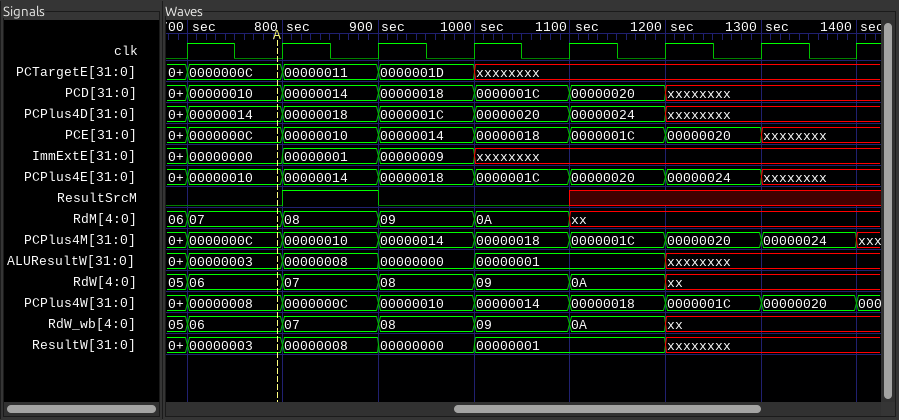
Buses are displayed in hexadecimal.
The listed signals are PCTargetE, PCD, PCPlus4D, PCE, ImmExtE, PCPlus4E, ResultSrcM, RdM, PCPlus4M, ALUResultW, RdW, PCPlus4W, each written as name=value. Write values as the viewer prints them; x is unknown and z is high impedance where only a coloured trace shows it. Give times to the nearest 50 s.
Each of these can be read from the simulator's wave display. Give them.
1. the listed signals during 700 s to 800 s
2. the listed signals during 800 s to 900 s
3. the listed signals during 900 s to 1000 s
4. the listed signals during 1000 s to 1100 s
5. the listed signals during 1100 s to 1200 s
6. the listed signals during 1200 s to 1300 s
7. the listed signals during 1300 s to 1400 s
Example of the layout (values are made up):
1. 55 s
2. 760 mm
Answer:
1. PCTargetE=0000000C, PCD=00000010, PCPlus4D=00000014, PCE=0000000C, ImmExtE=00000000, PCPlus4E=00000010, ResultSrcM=0, RdM=07, PCPlus4M=0000000C, ALUResultW=00000003, RdW=06, PCPlus4W=00000008
2. PCTargetE=00000011, PCD=00000014, PCPlus4D=00000018, PCE=00000010, ImmExtE=00000001, PCPlus4E=00000014, ResultSrcM=1, RdM=08, PCPlus4M=00000010, ALUResultW=00000008, RdW=07, PCPlus4W=0000000C
3. PCTargetE=0000001D, PCD=00000018, PCPlus4D=0000001C, PCE=00000014, ImmExtE=00000009, PCPlus4E=00000018, ResultSrcM=0, RdM=09, PCPlus4M=00000014, ALUResultW=00000000, RdW=08, PCPlus4W=00000010
4. PCTargetE=xxxxxxxx, PCD=0000001C, PCPlus4D=00000020, PCE=00000018, ImmExtE=xxxxxxxx, PCPlus4E=0000001C, ResultSrcM=0, RdM=0A, PCPlus4M=00000018, ALUResultW=00000001, RdW=09, PCPlus4W=00000014
5. PCTargetE=xxxxxxxx, PCD=00000020, PCPlus4D=00000024, PCE=0000001C, ImmExtE=xxxxxxxx, PCPlus4E=00000020, ResultSrcM=x, RdM=xx, PCPlus4M=0000001C, ALUResultW=00000001, RdW=0A, PCPlus4W=00000018
6. PCTargetE=xxxxxxxx, PCD=xxxxxxxx, PCPlus4D=xxxxxxxx, PCE=00000020, ImmExtE=xxxxxxxx, PCPlus4E=00000024, ResultSrcM=x, RdM=xx, PCPlus4M=00000020, ALUResultW=xxxxxxxx, RdW=xx, PCPlus4W=0000001C
7. PCTargetE=xxxxxxxx, PCD=xxxxxxxx, PCPlus4D=xxxxxxxx, PCE=xxxxxxxx, ImmExtE=xxxxxxxx, PCPlus4E=xxxxxxxx, ResultSrcM=x, RdM=xx, PCPlus4M=00000024, ALUResultW=xxxxxxxx, RdW=xx, PCPlus4W=00000020
